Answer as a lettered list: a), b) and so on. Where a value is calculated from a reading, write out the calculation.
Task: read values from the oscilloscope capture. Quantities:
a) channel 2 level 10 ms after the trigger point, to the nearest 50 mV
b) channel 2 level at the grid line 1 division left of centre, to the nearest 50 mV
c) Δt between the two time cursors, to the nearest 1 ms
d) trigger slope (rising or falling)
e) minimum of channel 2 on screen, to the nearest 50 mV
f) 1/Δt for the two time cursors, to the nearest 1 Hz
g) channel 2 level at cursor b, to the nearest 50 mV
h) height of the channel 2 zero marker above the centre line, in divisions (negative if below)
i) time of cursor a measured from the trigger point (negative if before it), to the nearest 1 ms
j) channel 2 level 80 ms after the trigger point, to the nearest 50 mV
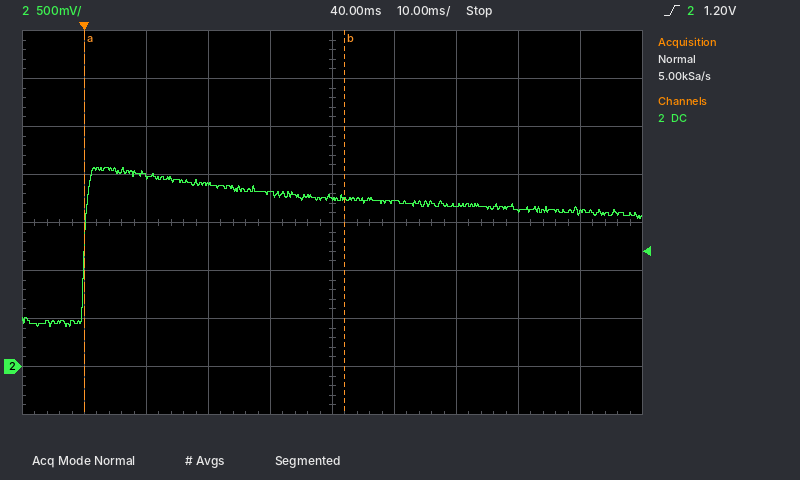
a) 2.00 V
b) 1.80 V
c) 42 ms
d) rising
e) 400 mV
f) 1 / 42 ms ≈ 24 Hz
g) 1.75 V
h) -3.0 div
i) 0 ms
j) 1.60 V
